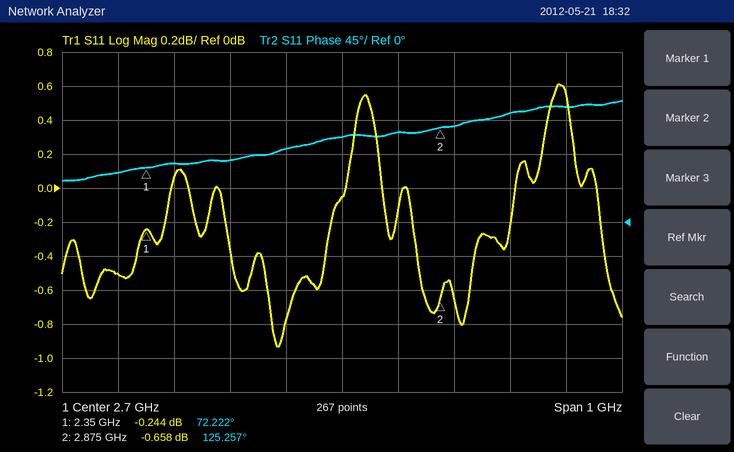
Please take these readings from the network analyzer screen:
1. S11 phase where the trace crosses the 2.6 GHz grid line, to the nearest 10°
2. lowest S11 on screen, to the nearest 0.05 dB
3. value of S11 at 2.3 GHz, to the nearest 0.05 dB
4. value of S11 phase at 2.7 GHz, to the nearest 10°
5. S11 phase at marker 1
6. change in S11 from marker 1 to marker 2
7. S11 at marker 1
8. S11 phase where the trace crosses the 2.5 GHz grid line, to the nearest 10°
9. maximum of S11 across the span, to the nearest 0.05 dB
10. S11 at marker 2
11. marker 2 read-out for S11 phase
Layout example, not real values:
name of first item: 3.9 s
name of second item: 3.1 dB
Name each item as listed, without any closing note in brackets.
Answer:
S11 phase where the trace crosses the 2.6 GHz grid line, to the nearest 10°: 100°
lowest S11 on screen, to the nearest 0.05 dB: -0.95 dB
value of S11 at 2.3 GHz, to the nearest 0.05 dB: -0.50 dB
value of S11 phase at 2.7 GHz, to the nearest 10°: 110°
S11 phase at marker 1: 72.222°
change in S11 from marker 1 to marker 2: -0.414 dB
S11 at marker 1: -0.244 dB
S11 phase where the trace crosses the 2.5 GHz grid line, to the nearest 10°: 80°
maximum of S11 across the span, to the nearest 0.05 dB: 0.60 dB
S11 at marker 2: -0.658 dB
marker 2 read-out for S11 phase: 125.257°
